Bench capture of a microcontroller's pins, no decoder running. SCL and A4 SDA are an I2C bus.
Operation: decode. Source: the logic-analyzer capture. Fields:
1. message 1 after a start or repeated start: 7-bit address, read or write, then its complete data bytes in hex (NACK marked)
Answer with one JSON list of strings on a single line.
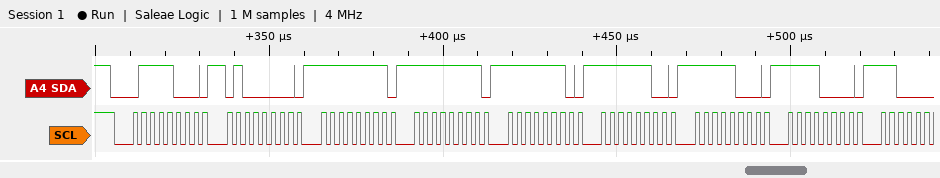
["0x3C write: 40 FF FF FE FC F8 F0"]
